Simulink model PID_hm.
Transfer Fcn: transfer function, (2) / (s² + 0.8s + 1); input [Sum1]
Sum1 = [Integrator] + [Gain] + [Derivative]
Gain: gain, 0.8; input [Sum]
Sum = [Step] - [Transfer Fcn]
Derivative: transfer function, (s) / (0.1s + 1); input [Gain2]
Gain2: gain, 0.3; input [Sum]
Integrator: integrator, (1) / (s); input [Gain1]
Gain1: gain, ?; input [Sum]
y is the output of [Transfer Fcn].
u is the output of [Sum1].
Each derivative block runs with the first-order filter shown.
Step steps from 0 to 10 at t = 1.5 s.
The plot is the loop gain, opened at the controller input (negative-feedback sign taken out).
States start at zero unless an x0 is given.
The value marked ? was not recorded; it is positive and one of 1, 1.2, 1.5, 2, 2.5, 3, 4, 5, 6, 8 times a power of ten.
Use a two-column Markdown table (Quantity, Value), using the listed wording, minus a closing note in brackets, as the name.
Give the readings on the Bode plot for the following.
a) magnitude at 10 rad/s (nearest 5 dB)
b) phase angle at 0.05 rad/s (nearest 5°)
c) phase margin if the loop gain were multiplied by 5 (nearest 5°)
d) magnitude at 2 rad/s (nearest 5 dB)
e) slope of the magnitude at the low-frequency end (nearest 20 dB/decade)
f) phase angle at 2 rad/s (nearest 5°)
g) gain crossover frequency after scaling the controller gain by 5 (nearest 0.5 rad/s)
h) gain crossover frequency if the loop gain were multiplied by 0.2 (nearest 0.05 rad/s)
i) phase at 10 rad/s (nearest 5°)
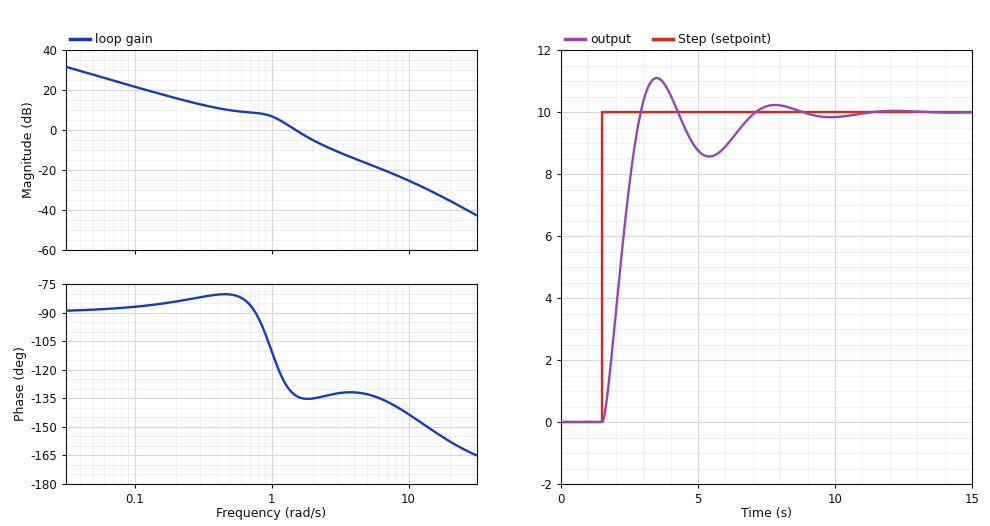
| Quantity | Value |
|---|---|
| magnitude at 10 rad/s | -25 dB |
| phase angle at 0.05 rad/s | -90° |
| phase margin if the loop gain were multiplied by 5 | 50° |
| magnitude at 2 rad/s | -5 dB |
| slope of the magnitude at the low-frequency end | -20 dB/decade |
| phase angle at 2 rad/s | -135° |
| gain crossover frequency after scaling the controller gain by 5 | 4.0 rad/s |
| gain crossover frequency if the loop gain were multiplied by 0.2 | 0.25 rad/s |
| phase at 10 rad/s | -145° |
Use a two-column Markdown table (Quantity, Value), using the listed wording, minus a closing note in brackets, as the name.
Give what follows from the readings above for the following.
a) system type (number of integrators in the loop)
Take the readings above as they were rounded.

| Quantity | Value |
|---|---|
| system type | 1 |
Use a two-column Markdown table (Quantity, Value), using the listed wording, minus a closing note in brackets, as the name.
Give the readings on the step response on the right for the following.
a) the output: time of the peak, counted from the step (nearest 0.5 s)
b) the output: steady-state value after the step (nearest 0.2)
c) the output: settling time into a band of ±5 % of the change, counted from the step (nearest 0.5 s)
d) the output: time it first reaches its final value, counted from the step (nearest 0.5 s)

| Quantity | Value |
|---|---|
| the output: time of the peak, counted from the step | 2.0 s |
| the output: steady-state value after the step | 10.0 |
| the output: settling time into a band of ±5 % of the change, counted from the step | 5.0 s |
| the output: time it first reaches its final value, counted from the step | 1.5 s |
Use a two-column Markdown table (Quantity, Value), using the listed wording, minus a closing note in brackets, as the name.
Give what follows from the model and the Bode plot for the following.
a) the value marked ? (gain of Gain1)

| Quantity | Value |
|---|---|
| the value marked ? | 0.6 |
